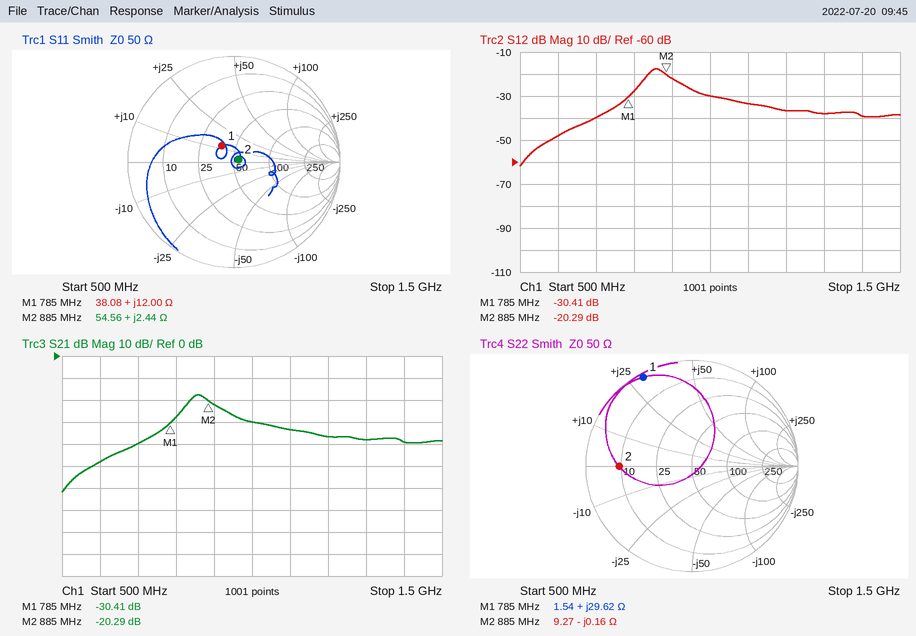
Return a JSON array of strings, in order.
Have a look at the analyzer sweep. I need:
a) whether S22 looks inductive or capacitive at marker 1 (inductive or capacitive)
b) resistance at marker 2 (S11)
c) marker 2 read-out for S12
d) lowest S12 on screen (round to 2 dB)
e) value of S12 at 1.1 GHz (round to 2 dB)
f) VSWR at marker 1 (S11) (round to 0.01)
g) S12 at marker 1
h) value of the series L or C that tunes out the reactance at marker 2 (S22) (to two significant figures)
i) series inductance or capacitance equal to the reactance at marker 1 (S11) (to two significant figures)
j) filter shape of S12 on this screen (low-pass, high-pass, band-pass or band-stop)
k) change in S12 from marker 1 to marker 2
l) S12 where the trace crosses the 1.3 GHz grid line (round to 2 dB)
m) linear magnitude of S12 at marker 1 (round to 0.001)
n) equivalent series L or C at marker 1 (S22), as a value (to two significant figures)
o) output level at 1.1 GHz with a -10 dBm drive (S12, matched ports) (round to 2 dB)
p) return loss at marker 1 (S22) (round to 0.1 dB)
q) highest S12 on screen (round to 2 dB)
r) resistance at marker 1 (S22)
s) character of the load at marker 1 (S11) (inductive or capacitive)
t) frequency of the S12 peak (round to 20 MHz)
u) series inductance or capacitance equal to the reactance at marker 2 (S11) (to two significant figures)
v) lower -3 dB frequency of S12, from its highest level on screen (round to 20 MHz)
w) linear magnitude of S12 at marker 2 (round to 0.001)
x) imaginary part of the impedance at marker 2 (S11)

["inductive", "54.56 Ω", "-20.29 dB", "-62 dB", "-34 dB", "1.47", "-30.41 dB", "29 pH", "2.4 nH", "band-pass", "10.12 dB", "-38 dB", "0.030", "6.0 nH", "-44 dBm", "0.4 dB", "-18 dB", "1.54 Ω", "inductive", "860 MHz", "440 pH", "840 MHz", "0.097", "+2.44 Ω"]
